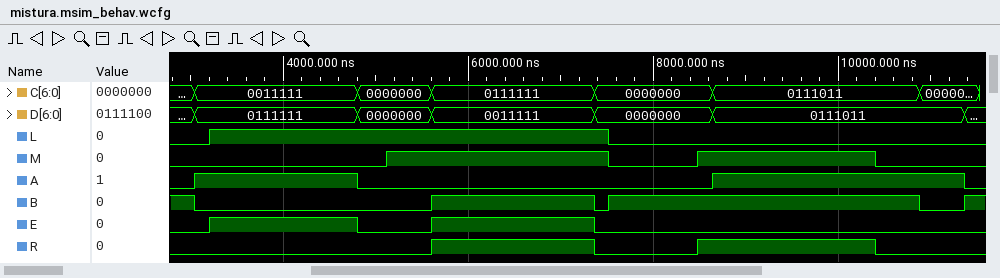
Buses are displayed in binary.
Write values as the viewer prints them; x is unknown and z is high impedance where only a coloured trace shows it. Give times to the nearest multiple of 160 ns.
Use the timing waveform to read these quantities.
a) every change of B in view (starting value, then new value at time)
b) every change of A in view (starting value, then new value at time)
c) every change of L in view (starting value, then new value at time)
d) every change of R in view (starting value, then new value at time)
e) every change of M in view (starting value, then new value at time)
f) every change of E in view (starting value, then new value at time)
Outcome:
1, 0 at 3040 ns, 1 at 5600 ns, 0 at 7360 ns, 1 at 7520 ns, 0 at 10880 ns, 1 at 11360 ns
0, 1 at 3040 ns, 0 at 4800 ns, 1 at 8640 ns, 0 at 11360 ns
0, 1 at 3200 ns, 0 at 7520 ns
0, 1 at 5600 ns, 0 at 7360 ns, 1 at 8480 ns, 0 at 10400 ns
0, 1 at 5120 ns, 0 at 7520 ns, 1 at 8480 ns, 0 at 10400 ns
0, 1 at 3200 ns, 0 at 4800 ns, 1 at 5600 ns, 0 at 7360 ns
